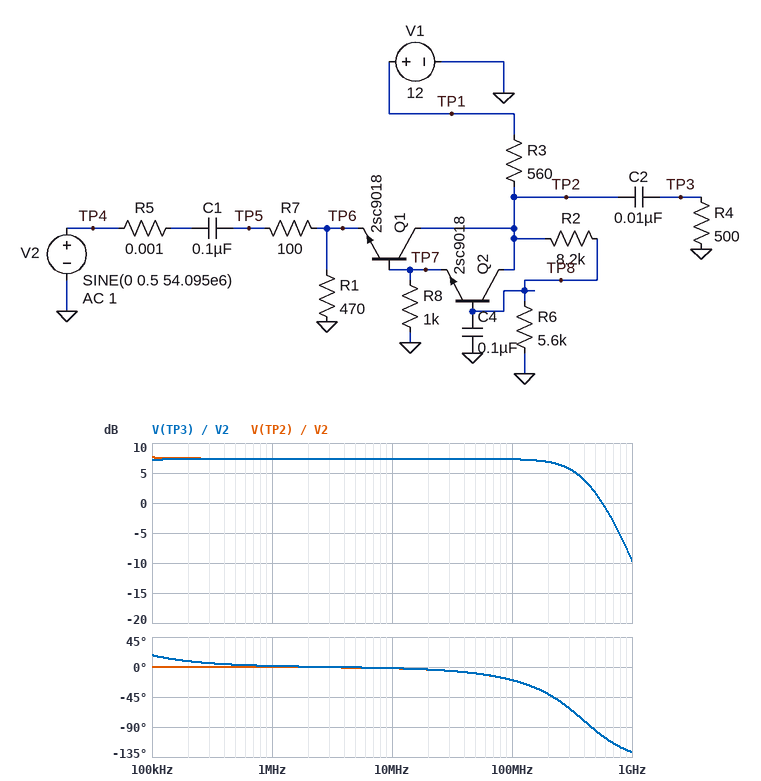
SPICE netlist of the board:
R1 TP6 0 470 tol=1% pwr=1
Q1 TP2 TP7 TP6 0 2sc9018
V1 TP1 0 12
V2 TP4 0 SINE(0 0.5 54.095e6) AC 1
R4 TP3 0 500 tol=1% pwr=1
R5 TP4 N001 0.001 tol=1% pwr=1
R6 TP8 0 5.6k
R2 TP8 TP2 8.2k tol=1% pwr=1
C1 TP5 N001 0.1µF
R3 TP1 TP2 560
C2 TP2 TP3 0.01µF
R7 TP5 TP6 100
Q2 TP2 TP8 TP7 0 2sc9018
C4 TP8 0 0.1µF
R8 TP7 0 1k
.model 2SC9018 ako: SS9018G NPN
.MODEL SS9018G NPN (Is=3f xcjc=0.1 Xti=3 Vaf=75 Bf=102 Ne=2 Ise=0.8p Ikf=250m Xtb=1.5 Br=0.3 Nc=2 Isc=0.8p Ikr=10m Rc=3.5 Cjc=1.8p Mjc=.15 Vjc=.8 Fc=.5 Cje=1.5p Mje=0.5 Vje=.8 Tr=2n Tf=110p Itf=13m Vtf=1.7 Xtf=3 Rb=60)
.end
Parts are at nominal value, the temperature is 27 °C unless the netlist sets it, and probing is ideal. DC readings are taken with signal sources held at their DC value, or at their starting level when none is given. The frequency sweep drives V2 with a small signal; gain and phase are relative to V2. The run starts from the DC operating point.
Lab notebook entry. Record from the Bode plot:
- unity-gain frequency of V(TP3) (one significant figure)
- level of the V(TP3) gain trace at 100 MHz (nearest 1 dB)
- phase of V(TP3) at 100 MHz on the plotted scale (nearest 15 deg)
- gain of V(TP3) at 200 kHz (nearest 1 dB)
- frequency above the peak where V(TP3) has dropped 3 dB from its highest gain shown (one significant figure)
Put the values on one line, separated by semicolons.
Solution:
600 MHz; 7 dB; -15 deg; 7 dB; 400 MHz
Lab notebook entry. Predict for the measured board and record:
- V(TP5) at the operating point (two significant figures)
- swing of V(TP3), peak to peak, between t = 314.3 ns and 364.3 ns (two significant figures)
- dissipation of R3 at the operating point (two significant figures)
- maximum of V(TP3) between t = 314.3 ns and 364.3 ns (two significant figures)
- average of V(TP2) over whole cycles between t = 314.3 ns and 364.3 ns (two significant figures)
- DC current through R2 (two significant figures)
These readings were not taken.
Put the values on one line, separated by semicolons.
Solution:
1.8 V; 2.2 V; 27 mW; 970 mV; 8.1 V; 600 µA
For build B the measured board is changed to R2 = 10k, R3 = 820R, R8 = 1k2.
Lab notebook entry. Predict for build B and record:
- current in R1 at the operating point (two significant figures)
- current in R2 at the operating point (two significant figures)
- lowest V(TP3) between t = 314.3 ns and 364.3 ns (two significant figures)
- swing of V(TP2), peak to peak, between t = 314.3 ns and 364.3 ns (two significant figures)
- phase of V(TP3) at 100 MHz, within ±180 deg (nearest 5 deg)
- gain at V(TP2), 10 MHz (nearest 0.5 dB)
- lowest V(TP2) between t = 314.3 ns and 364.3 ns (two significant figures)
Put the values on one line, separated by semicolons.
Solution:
2.9 mA; 510 µA; -1.4 V; 2.3 V; -25 deg; 8.5 dB; 6.5 V
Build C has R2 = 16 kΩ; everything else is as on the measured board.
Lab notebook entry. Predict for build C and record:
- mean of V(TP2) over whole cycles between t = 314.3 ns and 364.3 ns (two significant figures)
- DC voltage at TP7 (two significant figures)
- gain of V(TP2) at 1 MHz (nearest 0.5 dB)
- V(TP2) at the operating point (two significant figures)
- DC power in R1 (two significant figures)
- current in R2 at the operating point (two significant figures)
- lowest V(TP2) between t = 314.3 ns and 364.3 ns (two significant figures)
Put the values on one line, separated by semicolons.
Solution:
9.4 V; 1.7 V; 7.0 dB; 9.6 V; 2.2 mW; 450 µA; 8.4 V
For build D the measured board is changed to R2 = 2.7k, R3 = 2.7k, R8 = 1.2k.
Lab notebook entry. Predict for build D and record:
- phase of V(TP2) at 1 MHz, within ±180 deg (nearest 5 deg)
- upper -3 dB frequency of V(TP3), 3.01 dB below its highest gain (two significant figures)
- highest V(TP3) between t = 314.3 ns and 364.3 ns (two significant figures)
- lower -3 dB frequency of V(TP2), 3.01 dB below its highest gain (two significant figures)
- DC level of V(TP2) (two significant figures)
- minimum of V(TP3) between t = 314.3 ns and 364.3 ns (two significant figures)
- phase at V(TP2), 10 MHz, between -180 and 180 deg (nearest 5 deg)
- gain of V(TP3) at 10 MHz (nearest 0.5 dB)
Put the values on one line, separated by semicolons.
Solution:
0 deg; 220 MHz; 700 mV; 6.6 kHz; 3.2 V; -1.6 V; -5 deg; 9.5 dB
